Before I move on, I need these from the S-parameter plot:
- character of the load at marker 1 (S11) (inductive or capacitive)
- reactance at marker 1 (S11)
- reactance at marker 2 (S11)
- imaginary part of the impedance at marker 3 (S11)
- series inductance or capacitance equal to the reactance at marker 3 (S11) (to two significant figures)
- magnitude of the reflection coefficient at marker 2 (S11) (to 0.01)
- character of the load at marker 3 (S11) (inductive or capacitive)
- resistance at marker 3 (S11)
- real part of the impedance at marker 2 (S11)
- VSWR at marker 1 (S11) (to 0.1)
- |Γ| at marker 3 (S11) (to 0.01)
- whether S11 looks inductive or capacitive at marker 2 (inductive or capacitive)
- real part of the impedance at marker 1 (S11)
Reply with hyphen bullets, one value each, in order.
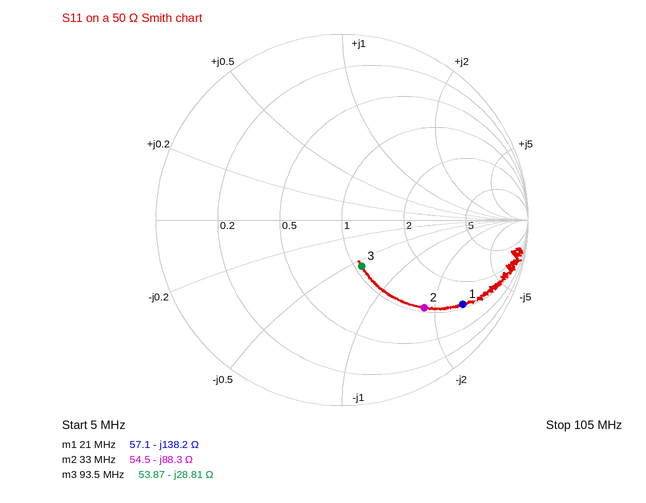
- capacitive
- -138.2 Ω
- -88.3 Ω
- -28.81 Ω
- 59 pF
- 0.65
- capacitive
- 53.87 Ω
- 54.5 Ω
- 8.6
- 0.27
- capacitive
- 57.1 Ω
